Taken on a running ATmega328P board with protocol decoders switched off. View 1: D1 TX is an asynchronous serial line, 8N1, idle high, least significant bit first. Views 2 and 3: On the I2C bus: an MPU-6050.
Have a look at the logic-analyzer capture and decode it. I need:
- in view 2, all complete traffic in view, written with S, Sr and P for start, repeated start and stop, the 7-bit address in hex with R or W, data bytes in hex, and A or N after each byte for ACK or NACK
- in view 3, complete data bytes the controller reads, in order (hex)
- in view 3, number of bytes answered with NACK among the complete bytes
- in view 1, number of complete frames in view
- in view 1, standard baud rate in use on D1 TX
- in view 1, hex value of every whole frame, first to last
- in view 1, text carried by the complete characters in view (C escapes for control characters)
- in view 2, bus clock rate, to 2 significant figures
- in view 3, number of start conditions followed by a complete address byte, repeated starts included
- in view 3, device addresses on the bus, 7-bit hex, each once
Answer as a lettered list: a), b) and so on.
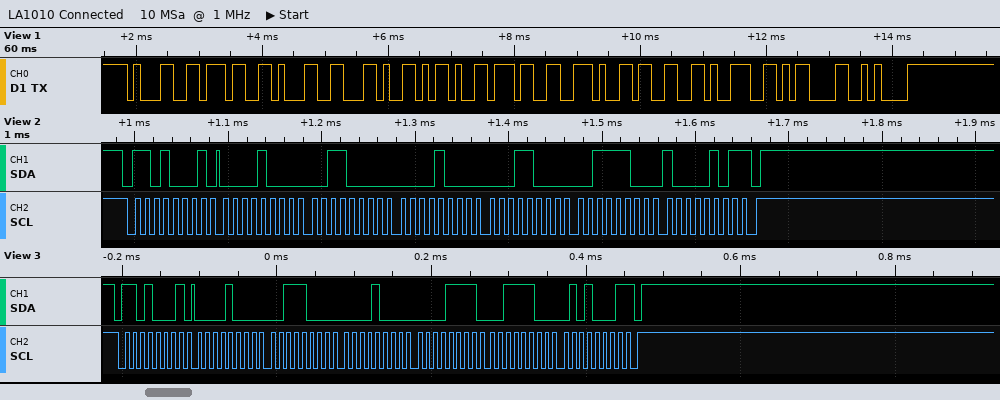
a) S 68R A 08 A 30 A 08 A 18 A 3C A 85 N P
b) 08 38 08 0F 3C 51
c) 1
d) 11
e) 9600 baud
f) 31 37 31 2C 2D 37 2E 33 39 0D 0A
g) "171,-7.39\r\n"
h) 100 kHz
i) 1
j) 0x68
